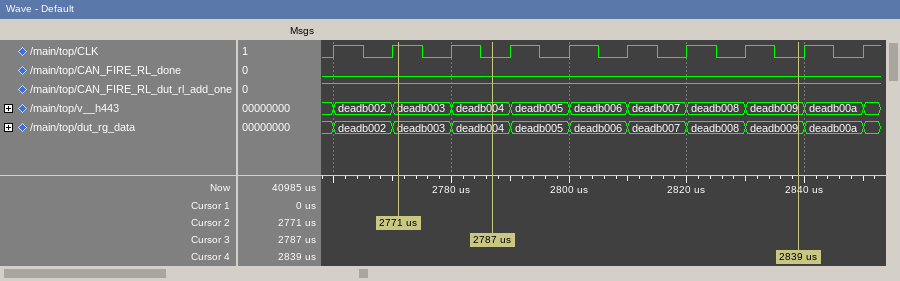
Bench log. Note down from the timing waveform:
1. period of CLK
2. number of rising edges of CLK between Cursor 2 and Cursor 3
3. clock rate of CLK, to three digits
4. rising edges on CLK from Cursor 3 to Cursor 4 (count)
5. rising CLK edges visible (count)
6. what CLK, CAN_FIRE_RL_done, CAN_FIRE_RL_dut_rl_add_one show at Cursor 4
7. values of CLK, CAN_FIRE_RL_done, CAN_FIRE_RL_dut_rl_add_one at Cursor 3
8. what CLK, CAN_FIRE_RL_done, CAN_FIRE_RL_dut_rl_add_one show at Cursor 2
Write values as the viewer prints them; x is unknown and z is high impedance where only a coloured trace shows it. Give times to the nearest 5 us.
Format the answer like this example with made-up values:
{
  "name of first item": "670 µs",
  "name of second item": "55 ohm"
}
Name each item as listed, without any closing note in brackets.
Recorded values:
{
  "period of CLK": "10 us",
  "number of rising edges of CLK between Cursor 2 and Cursor 3": "1",
  "clock rate of CLK, to three digits": "100 kHz",
  "rising edges on CLK from Cursor 3 to Cursor 4": "5",
  "rising CLK edges visible": "10",
  "what CLK, CAN_FIRE_RL_done, CAN_FIRE_RL_dut_rl_add_one show at Cursor 4": "CLK=0, CAN_FIRE_RL_done=0, CAN_FIRE_RL_dut_rl_add_one=1",
  "values of CLK, CAN_FIRE_RL_done, CAN_FIRE_RL_dut_rl_add_one at Cursor 3": "CLK=0, CAN_FIRE_RL_done=0, CAN_FIRE_RL_dut_rl_add_one=1",
  "what CLK, CAN_FIRE_RL_done, CAN_FIRE_RL_dut_rl_add_one show at Cursor 2": "CLK=1, CAN_FIRE_RL_done=0, CAN_FIRE_RL_dut_rl_add_one=1"
}
